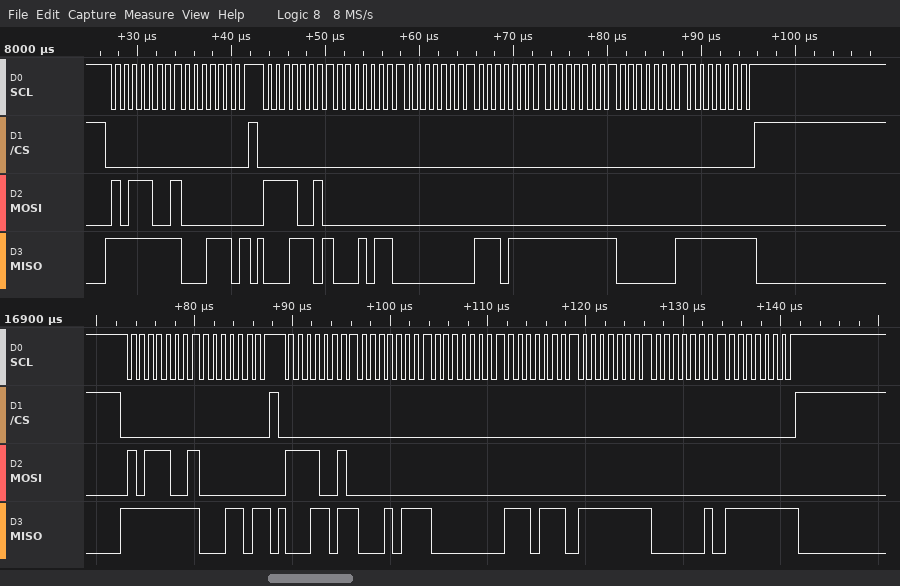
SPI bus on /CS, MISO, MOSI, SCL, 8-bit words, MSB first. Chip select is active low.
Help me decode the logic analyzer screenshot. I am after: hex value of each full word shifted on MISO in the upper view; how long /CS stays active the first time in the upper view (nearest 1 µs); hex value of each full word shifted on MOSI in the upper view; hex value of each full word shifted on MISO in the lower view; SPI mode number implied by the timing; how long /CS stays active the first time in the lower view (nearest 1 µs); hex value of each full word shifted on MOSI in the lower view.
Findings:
FF, 1D, 1D, 16, 00, EF, FF, 01, FF
15 µs
B9, 00, F2, 00, 00, 00, 00, 00, 00
FF, 1B, 1B, 17, 00, EE, FF, 02, FF
3
15 µs
B9, 00, F2, 00, 00, 00, 00, 00, 00
